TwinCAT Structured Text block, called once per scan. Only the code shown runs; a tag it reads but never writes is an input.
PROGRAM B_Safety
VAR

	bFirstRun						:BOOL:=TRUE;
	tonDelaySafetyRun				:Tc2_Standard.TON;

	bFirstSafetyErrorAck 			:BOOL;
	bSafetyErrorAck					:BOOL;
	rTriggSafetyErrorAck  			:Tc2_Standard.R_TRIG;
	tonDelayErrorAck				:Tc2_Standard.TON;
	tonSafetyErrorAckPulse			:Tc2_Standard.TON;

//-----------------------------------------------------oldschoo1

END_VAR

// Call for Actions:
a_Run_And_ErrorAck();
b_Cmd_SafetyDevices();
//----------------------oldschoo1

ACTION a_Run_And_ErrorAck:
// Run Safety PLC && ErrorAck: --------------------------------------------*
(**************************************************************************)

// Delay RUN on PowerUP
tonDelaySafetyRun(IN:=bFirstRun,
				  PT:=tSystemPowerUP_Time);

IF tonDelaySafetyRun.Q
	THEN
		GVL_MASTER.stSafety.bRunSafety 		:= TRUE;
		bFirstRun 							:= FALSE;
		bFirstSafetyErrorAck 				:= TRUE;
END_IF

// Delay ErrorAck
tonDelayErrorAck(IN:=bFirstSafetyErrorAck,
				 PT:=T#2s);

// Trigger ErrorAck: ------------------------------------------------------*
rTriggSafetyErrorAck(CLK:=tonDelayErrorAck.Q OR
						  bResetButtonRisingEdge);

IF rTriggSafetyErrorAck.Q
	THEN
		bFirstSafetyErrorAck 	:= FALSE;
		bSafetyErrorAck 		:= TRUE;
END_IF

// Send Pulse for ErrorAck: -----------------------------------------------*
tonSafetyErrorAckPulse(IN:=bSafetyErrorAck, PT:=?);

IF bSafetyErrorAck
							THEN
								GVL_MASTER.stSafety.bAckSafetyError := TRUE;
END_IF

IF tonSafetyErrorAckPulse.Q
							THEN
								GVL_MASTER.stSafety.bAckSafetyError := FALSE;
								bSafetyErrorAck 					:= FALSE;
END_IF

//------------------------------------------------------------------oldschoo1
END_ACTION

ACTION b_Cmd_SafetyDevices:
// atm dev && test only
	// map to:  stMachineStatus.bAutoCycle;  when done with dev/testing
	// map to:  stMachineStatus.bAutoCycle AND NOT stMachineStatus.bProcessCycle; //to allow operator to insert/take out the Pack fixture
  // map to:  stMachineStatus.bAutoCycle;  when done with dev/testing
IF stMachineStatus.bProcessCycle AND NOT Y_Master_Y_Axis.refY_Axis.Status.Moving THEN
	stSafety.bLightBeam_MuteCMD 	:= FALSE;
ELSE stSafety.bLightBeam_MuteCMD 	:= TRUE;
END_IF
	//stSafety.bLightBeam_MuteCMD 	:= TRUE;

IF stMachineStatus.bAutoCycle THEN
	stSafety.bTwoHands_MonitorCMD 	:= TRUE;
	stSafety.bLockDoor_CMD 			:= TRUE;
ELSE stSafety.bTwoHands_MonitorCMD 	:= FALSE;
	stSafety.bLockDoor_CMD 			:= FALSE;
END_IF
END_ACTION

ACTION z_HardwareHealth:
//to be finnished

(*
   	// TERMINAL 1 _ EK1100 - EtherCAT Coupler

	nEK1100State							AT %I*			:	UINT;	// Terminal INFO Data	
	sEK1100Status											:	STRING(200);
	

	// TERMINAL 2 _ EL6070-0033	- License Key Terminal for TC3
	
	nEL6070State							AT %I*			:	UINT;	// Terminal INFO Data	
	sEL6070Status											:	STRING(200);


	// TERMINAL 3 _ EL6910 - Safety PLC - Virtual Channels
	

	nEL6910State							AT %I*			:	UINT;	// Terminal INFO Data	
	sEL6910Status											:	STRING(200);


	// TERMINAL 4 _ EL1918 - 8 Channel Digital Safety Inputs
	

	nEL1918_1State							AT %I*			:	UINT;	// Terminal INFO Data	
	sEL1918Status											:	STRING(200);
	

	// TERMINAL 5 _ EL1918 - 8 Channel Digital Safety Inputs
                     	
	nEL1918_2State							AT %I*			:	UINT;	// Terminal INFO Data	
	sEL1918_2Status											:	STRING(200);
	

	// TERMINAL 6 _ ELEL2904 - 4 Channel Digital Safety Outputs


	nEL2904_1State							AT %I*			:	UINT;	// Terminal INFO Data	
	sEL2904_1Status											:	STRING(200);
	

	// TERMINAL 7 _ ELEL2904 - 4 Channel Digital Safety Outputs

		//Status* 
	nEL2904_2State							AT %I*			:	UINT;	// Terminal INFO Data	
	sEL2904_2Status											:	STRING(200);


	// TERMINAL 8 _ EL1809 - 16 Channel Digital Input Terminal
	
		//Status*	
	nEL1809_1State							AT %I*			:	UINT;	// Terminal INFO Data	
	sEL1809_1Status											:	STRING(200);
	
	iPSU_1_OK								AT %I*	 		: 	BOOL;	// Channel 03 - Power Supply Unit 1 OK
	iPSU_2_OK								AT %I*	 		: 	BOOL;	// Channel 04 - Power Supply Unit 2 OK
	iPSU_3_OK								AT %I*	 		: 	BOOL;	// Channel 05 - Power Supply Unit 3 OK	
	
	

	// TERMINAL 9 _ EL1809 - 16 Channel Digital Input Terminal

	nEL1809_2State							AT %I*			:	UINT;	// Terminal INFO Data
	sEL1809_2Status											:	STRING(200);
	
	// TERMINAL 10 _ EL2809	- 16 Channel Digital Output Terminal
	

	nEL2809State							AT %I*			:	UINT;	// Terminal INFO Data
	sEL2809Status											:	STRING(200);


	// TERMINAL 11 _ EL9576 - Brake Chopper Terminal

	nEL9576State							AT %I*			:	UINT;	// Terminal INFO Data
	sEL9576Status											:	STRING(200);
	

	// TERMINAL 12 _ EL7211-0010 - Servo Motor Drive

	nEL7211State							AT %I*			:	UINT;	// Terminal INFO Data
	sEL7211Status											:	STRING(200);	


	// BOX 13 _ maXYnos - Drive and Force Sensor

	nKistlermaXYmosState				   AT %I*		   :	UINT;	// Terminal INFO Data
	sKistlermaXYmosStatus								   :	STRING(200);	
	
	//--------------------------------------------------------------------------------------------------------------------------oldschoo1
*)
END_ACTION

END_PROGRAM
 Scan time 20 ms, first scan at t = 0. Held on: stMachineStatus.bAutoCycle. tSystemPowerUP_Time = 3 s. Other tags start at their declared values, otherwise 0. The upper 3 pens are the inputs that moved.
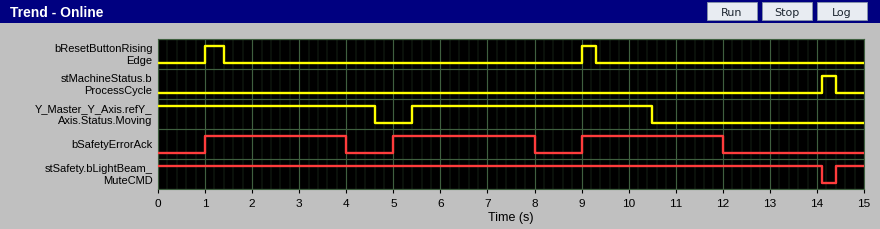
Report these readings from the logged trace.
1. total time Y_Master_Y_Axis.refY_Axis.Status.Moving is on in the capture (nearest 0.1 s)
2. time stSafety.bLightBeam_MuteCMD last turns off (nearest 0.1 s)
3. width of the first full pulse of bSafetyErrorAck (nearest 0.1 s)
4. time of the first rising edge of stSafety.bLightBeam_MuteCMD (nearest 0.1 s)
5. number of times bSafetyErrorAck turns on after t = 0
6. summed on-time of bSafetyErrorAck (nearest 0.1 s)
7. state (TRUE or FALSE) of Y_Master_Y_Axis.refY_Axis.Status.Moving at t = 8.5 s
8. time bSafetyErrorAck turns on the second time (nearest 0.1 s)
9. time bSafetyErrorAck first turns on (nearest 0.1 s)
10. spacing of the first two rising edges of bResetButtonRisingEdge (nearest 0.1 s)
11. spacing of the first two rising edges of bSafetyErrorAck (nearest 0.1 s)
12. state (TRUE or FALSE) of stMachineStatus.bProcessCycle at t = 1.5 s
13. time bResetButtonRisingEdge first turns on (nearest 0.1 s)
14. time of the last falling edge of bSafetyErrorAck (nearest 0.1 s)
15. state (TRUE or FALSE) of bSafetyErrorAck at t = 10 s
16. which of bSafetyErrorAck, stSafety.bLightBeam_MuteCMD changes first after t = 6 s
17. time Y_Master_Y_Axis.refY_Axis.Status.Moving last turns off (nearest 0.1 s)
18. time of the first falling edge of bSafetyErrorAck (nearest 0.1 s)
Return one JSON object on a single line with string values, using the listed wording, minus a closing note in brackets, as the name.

{"total time Y_Master_Y_Axis.refY_Axis.Status.Moving is on in the capture": "9.7 s", "time stSafety.bLightBeam_MuteCMD last turns off": "14.1 s", "width of the first full pulse of bSafetyErrorAck": "3.0 s", "time of the first rising edge of stSafety.bLightBeam_MuteCMD": "14.4 s", "number of times bSafetyErrorAck turns on after t = 0": "3", "summed on-time of bSafetyErrorAck": "9.0 s", "state (TRUE or FALSE) of Y_Master_Y_Axis.refY_Axis.Status.Moving at t = 8.5 s": "TRUE", "time bSafetyErrorAck turns on the second time": "5.0 s", "time bSafetyErrorAck first turns on": "1.0 s", "spacing of the first two rising edges of bResetButtonRisingEdge": "8.0 s", "spacing of the first two rising edges of bSafetyErrorAck": "4.0 s", "state (TRUE or FALSE) of stMachineStatus.bProcessCycle at t = 1.5 s": "FALSE", "time bResetButtonRisingEdge first turns on": "1.0 s", "time of the last falling edge of bSafetyErrorAck": "12.0 s", "state (TRUE or FALSE) of bSafetyErrorAck at t = 10 s": "TRUE", "which of bSafetyErrorAck, stSafety.bLightBeam_MuteCMD changes first after t = 6 s": "bSafetyErrorAck", "time Y_Master_Y_Axis.refY_Axis.Status.Moving last turns off": "10.5 s", "time of the first falling edge of bSafetyErrorAck": "4.0 s"}
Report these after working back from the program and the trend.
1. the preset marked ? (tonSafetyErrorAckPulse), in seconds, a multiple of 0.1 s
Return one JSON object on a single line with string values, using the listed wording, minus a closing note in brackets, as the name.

{"the preset marked ? (tonSafetyErrorAckPulse), in seconds, a multiple of 0.1 s": "3.0 s"}
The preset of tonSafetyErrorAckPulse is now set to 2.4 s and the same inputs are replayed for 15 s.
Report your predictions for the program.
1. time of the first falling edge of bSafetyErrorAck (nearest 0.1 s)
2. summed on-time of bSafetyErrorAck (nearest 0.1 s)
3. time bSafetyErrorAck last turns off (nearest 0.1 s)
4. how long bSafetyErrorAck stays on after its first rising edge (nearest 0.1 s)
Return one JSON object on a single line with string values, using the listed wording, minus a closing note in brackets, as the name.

{"time of the first falling edge of bSafetyErrorAck": "3.4 s", "summed on-time of bSafetyErrorAck": "7.2 s", "time bSafetyErrorAck last turns off": "11.4 s", "how long bSafetyErrorAck stays on after its first rising edge": "2.4 s"}
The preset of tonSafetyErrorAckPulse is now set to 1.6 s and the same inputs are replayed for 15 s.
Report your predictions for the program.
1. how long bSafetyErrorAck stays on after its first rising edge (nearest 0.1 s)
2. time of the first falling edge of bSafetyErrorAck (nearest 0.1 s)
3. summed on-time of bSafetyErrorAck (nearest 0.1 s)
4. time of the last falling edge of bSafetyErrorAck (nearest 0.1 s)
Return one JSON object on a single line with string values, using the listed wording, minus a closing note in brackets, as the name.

{"how long bSafetyErrorAck stays on after its first rising edge": "1.6 s", "time of the first falling edge of bSafetyErrorAck": "2.6 s", "summed on-time of bSafetyErrorAck": "4.8 s", "time of the last falling edge of bSafetyErrorAck": "10.6 s"}
